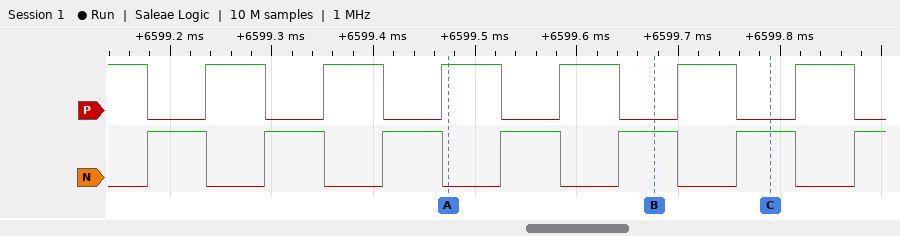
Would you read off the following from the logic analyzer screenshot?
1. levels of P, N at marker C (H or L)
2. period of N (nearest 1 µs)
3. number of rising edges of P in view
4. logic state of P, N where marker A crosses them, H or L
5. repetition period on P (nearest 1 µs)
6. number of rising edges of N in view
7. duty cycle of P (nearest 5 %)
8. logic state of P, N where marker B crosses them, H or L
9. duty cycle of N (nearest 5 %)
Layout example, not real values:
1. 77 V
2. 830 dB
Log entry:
1. P=L, N=H
2. 116 µs
3. 6
4. P=H, N=L
5. 116 µs
6. 7
7. 50 %
8. P=L, N=H
9. 50 %
